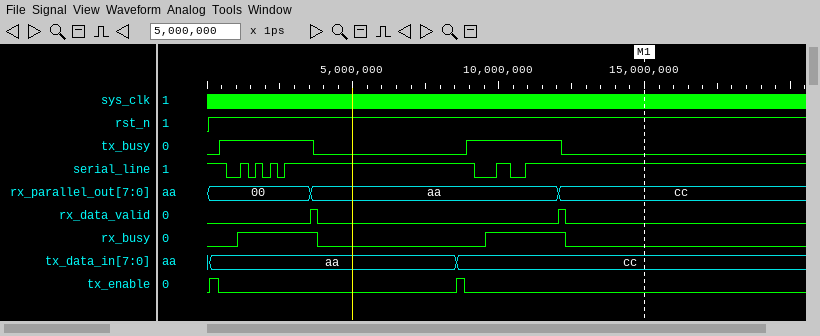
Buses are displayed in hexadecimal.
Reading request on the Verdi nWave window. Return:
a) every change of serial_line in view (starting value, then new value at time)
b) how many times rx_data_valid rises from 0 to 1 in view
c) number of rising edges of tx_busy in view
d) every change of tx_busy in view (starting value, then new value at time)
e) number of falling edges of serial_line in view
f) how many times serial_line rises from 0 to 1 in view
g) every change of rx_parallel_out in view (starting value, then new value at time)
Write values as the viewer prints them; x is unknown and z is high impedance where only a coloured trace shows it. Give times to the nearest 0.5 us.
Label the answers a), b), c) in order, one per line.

a) 1, 0 at 0.5 us, 1 at 1 us, 0 at 1.5 us, 1 at 1.5 us, 0 at 2 us, 1 at 2 us, 0 at 2.5 us, 1 at 2.5 us, 0 at 9 us, 1 at 10 us, 0 at 10.5 us, 1 at 11 us
b) 2
c) 2
d) 0, 1 at 0.5 us, 0 at 3.5 us, 1 at 9 us, 0 at 12 us
e) 6
f) 6
g) 00, aa at 3.5 us, cc at 12 us
